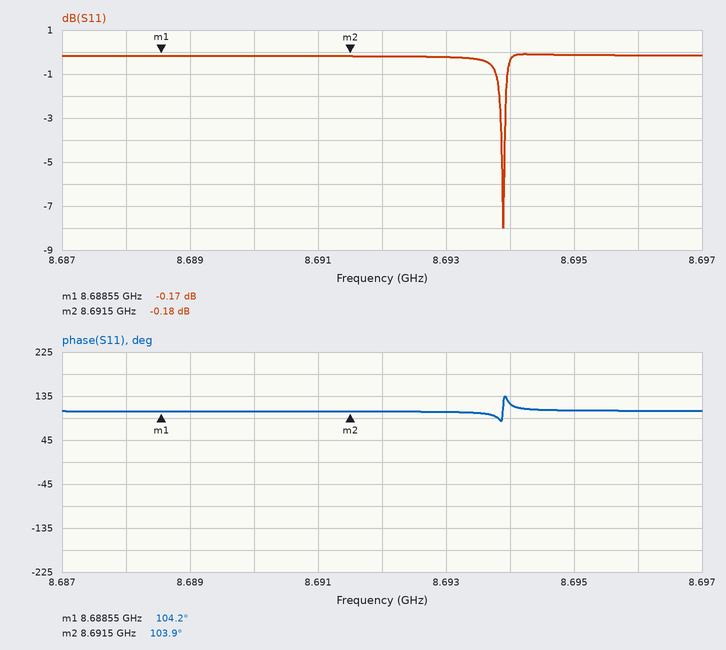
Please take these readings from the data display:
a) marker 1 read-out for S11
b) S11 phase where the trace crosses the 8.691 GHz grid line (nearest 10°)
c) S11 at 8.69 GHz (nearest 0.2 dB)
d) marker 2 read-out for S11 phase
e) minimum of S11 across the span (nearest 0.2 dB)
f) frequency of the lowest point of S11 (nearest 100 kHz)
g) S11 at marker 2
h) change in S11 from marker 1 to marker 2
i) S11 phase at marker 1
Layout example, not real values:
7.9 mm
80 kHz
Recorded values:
-0.17 dB
100°
-0.2 dB
103.9°
-8.0 dB
8.6939 GHz
-0.18 dB
-0.01 dB
104.2°
